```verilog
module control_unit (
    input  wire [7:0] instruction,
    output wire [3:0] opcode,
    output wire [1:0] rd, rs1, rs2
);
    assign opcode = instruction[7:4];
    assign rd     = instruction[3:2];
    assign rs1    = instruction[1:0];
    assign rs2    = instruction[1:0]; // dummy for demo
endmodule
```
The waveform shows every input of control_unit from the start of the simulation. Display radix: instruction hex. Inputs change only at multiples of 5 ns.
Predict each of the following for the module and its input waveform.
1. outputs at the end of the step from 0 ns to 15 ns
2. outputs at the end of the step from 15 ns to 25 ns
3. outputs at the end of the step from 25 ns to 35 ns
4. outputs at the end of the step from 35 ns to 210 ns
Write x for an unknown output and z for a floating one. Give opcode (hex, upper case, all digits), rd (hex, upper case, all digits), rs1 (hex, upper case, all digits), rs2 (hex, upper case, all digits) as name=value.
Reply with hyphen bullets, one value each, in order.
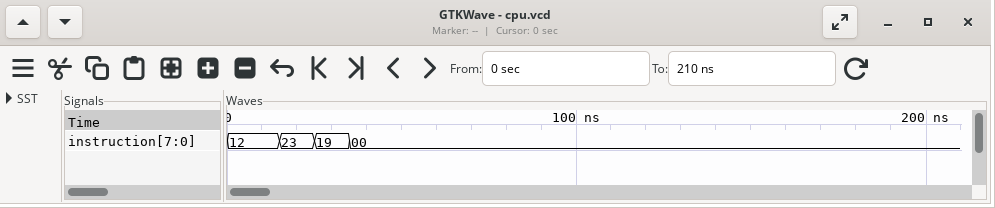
- opcode=1, rd=0, rs1=2, rs2=2
- opcode=2, rd=0, rs1=3, rs2=3
- opcode=1, rd=2, rs1=1, rs2=1
- opcode=0, rd=0, rs1=0, rs2=0
